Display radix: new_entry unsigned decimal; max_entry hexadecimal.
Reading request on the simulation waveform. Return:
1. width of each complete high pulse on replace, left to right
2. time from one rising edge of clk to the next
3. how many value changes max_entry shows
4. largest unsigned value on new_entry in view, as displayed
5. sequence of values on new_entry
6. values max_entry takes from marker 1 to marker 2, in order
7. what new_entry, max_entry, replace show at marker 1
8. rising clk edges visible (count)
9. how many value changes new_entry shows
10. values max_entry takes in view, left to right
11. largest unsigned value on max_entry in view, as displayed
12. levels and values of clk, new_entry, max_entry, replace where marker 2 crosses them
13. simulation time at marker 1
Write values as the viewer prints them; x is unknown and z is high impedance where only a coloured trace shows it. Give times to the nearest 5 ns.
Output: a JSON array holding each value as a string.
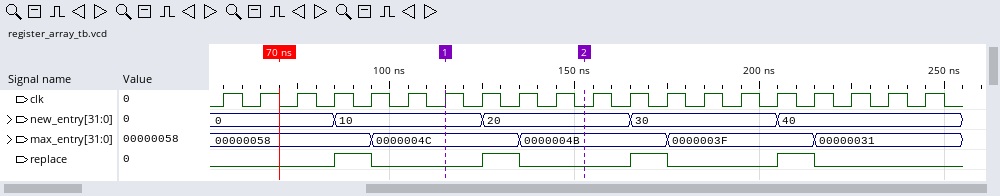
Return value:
["10 ns, 10 ns, 10 ns, 10 ns", "10 ns", "4", "40", "0, 10, 20, 30, 40", "0000004C, 0000004B", "new_entry=10, max_entry=0000004C, replace=0", "20", "4", "00000058, 0000004C, 0000004B, 0000003F, 00000031", "00000058", "clk=0, new_entry=20, max_entry=0000004B, replace=0", "115 ns"]
